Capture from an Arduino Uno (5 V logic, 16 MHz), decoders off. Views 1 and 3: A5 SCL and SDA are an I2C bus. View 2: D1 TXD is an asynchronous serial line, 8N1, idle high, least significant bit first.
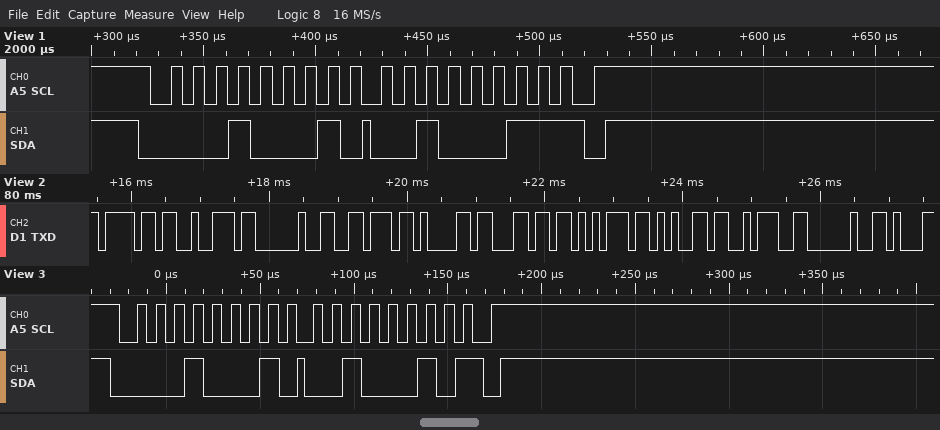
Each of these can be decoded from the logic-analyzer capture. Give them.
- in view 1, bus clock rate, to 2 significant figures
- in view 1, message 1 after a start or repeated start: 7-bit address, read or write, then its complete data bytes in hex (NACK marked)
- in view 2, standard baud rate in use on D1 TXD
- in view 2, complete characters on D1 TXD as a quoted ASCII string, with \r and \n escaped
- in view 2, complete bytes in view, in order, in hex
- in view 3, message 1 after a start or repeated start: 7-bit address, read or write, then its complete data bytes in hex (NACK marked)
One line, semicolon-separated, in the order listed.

100 kHz; 0x08 read: 23 NACK; 9600 baud; "or value: "; 6F 72 20 76 61 6C 75 65 3A 20; 0x08 read: 22 NACK
